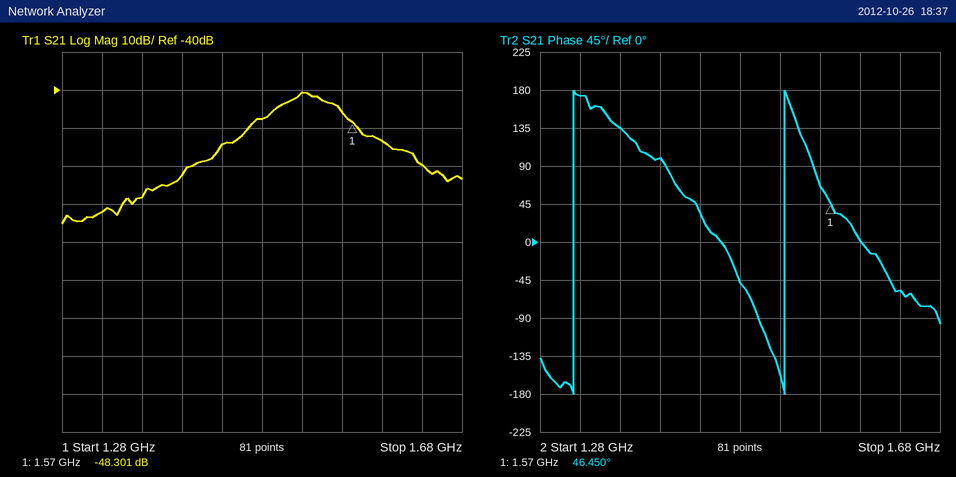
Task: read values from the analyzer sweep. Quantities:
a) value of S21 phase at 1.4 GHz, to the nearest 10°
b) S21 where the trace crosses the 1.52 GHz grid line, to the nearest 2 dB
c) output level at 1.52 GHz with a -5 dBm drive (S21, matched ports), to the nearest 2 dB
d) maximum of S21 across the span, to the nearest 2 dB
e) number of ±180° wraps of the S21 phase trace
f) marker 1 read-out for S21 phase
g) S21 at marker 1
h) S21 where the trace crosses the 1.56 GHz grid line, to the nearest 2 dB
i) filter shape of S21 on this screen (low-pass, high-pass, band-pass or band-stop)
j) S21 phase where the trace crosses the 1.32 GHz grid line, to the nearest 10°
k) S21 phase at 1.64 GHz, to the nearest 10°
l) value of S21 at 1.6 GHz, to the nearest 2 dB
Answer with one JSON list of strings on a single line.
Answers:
["100°", "-40 dB", "-46 dBm", "-40 dB", "2", "46.450°", "-48.301 dB", "-46 dB", "band-pass", "170°", "-60°", "-54 dB"]
